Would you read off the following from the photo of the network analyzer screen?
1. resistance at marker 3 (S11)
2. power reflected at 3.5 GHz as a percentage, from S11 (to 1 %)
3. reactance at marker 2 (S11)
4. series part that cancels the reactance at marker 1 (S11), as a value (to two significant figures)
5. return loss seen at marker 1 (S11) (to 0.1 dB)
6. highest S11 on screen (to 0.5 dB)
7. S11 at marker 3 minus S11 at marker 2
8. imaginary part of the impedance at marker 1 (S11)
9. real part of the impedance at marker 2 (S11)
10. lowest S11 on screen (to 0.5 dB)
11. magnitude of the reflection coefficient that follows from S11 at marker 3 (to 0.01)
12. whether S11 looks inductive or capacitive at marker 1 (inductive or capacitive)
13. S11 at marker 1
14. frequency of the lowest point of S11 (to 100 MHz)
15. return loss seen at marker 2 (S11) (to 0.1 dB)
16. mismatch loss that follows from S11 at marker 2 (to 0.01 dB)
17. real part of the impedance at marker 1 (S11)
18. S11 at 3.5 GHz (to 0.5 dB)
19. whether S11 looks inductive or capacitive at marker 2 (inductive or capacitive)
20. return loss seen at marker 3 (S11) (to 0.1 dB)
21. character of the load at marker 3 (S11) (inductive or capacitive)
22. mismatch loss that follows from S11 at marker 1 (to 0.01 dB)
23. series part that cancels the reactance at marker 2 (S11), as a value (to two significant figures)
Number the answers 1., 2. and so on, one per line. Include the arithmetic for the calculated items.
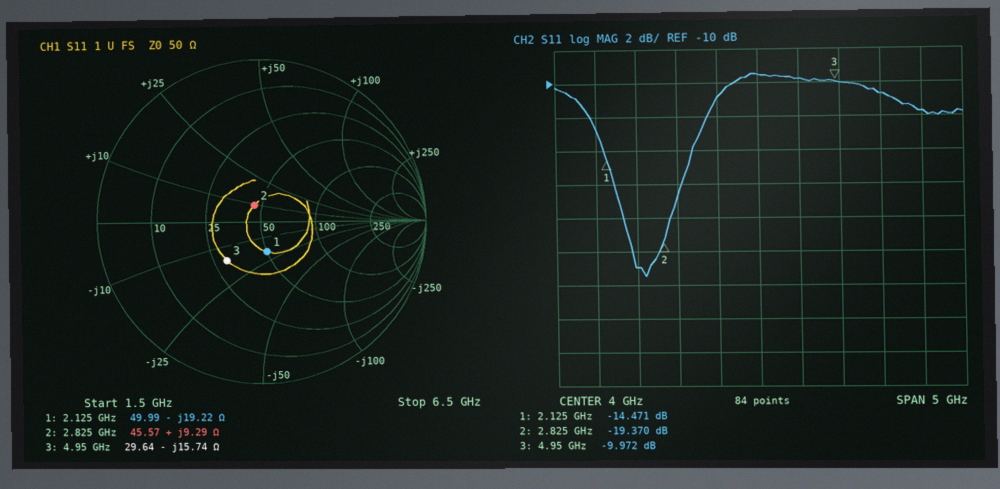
1. 29.64 Ω
2. 10^(-11/10) ≈ 8 %
3. +9.29 Ω
4. L = 19.22 Ω/(2π × 2.125 GHz) ≈ 1.4 nH
5. 14.5 dB
6. -9.5 dB
7. -9.972 − (-19.37) = 9.398 dB
8. -19.22 Ω
9. 45.57 Ω
10. -21.5 dB
11. 10^(-9.972/20) ≈ 0.32
12. capacitive
13. -14.471 dB
14. 2.6 GHz
15. 19.4 dB
16. −10 log10(1 − 10^(-19.37/10)) ≈ 0.05 dB
17. 49.99 Ω
18. -11.0 dB
19. inductive
20. 10.0 dB
21. capacitive
22. −10 log10(1 − 10^(-14.471/10)) ≈ 0.16 dB
23. C = 1/(2π × 2.825 GHz × 9.29 Ω) ≈ 6.1 pF
